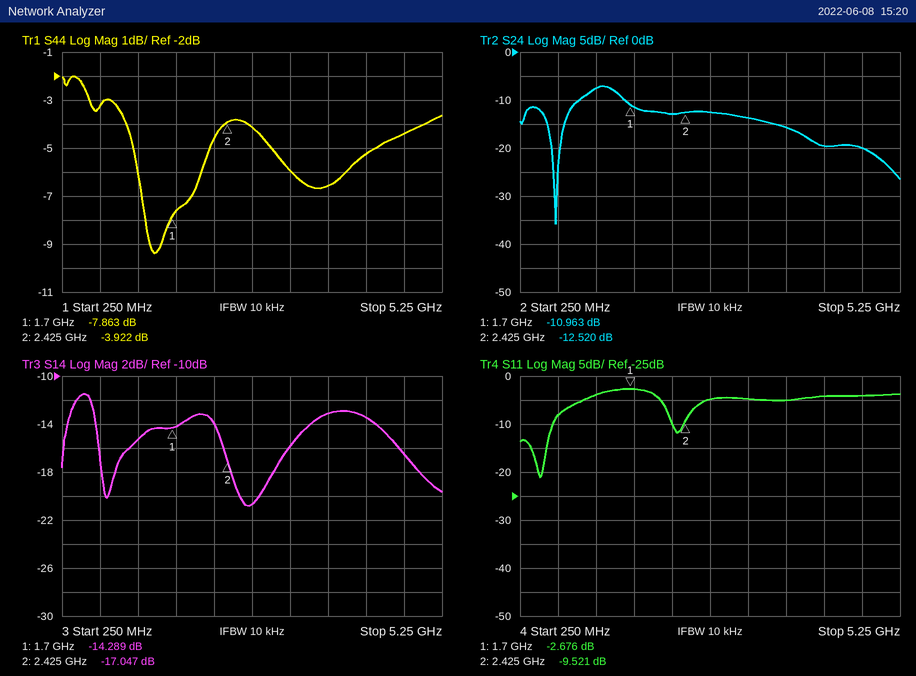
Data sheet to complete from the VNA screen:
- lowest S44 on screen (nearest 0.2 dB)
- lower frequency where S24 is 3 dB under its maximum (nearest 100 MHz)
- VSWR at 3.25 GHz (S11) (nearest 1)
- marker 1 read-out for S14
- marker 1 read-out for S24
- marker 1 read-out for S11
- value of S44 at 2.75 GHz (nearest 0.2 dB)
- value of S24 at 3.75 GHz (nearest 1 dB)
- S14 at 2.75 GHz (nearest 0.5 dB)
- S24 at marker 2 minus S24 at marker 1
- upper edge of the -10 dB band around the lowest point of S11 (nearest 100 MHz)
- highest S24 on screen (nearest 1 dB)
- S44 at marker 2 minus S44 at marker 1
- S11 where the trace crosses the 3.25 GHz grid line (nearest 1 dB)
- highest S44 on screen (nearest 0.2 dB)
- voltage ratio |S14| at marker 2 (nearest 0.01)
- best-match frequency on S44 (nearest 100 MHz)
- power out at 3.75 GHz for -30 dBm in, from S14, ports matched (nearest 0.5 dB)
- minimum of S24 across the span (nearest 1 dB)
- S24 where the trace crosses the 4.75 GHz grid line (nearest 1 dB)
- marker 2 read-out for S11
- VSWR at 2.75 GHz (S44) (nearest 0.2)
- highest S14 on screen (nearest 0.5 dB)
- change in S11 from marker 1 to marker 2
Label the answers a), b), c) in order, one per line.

a) -9.4 dB
b) 1.0 GHz
c) 4
d) -14.289 dB
e) -10.963 dB
f) -2.676 dB
g) -4.2 dB
h) -16 dB
i) -20.5 dB
j) -1.557 dB
k) 700 MHz
l) -7 dB
m) 3.941 dB
n) -5 dB
o) -2.0 dB
p) 0.14
q) 1.5 GHz
r) -43.0 dBm
s) -36 dB
t) -20 dB
u) -9.521 dB
v) 4.2
w) -11.5 dB
x) -6.845 dB
